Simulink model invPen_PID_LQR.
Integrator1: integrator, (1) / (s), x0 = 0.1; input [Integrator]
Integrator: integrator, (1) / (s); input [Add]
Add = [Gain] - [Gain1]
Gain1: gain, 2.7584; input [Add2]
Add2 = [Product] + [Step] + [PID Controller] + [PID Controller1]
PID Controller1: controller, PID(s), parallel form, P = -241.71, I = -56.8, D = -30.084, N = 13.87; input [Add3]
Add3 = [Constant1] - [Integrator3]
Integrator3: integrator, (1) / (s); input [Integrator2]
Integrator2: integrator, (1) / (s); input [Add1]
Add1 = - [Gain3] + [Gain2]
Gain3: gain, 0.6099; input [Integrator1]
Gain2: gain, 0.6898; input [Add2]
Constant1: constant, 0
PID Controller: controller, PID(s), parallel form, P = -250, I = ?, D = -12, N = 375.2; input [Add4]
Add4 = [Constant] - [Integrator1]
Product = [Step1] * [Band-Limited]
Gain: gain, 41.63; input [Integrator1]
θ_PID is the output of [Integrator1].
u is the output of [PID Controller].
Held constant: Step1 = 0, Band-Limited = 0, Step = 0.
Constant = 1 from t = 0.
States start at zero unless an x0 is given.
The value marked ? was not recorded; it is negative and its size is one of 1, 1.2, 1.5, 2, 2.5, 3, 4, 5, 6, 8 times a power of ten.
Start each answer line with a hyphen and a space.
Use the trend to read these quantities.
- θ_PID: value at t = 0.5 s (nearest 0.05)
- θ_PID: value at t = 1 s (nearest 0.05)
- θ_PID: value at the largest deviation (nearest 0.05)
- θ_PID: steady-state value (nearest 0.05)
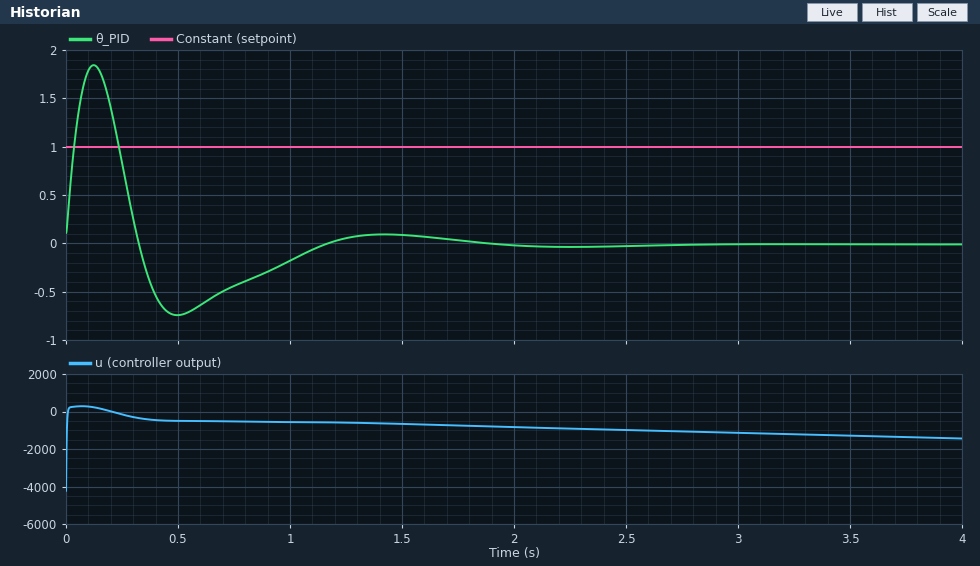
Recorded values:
- -0.75
- -0.20
- 1.85
- 0.00
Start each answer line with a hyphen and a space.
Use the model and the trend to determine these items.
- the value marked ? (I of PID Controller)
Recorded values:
- -300
